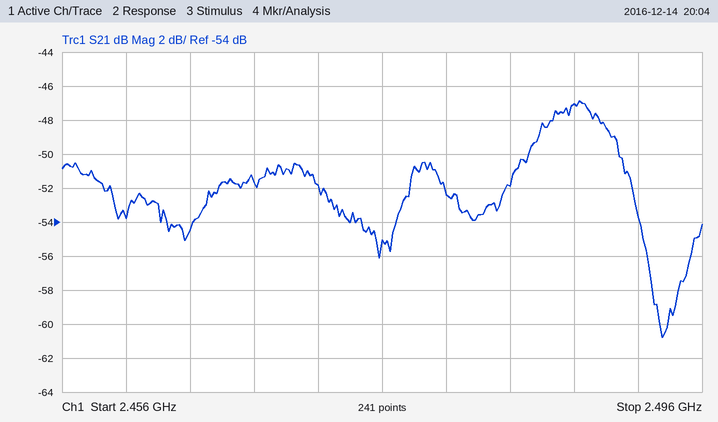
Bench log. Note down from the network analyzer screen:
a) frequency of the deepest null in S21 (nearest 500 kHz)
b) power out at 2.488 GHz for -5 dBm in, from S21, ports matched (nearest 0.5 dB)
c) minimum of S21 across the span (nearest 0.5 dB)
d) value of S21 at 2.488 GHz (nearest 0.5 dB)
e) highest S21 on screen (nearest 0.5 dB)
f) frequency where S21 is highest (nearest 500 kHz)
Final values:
2.4935 GHz
-52.0 dBm
-61.0 dB
-47.0 dB
-47.0 dB
2.4885 GHz
